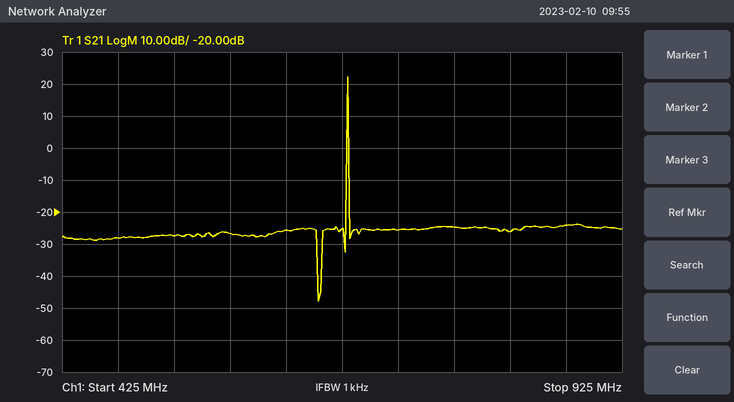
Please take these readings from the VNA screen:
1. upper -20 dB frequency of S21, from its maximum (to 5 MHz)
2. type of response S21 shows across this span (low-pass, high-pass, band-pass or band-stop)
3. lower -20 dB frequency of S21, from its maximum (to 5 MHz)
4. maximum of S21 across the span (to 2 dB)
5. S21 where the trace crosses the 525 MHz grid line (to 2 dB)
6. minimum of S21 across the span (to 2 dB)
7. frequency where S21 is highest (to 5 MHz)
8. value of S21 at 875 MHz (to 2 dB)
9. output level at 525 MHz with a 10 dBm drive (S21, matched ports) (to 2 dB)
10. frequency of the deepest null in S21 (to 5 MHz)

680 MHz
band-pass
680 MHz
22 dB
-28 dB
-48 dB
680 MHz
-24 dB
-18 dBm
655 MHz
